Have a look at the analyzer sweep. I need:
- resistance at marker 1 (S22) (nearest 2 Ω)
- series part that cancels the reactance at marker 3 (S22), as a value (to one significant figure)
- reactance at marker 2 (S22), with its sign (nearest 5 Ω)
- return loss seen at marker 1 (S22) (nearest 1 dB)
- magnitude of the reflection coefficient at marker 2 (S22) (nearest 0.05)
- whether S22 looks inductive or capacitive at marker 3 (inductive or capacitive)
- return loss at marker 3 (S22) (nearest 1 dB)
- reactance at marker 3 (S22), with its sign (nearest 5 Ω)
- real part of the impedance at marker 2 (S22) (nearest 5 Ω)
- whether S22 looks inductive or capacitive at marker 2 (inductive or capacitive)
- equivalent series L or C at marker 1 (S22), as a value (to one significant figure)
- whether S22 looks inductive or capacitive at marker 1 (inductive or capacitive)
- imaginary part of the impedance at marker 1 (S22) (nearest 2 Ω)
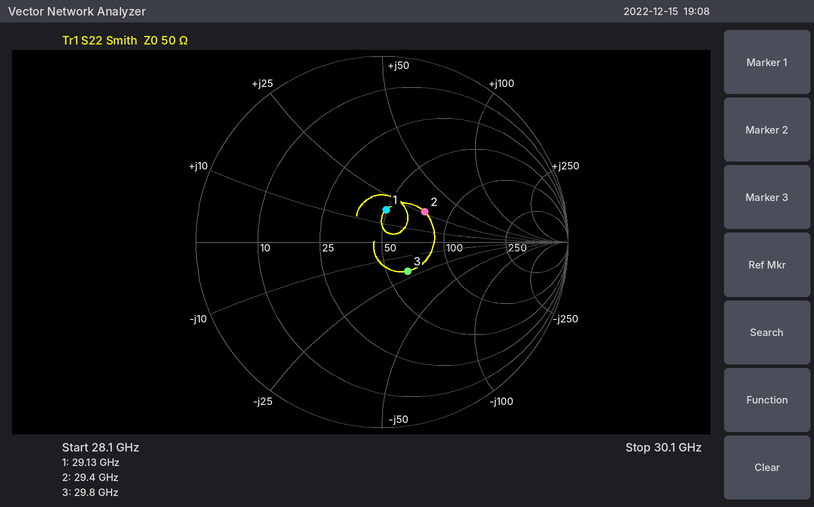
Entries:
50 Ω
100 pH
+25 Ω
15 dB
0.30
capacitive
14 dB
-20 Ω
75 Ω
inductive
100 pH
inductive
+18 Ω
